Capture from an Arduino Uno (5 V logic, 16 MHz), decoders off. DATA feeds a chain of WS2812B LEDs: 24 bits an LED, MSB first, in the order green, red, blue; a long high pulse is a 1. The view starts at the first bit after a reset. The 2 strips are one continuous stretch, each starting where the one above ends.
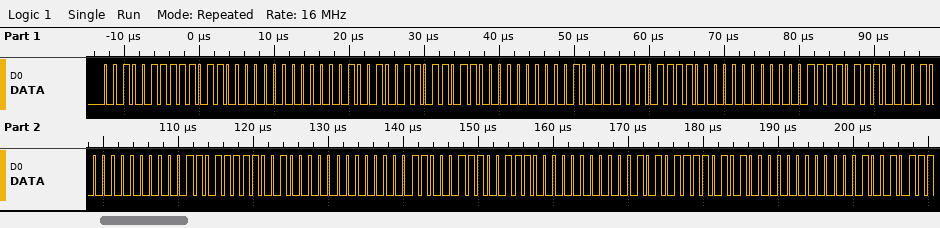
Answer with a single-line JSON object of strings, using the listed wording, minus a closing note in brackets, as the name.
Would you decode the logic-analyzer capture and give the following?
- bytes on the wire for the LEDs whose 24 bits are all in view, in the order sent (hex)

{"bytes on the wire for the LEDs whose 24 bits are all in view, in the order sent": "27 D8 00 24 DB 00 21 DE 00 1E E1 00 1B E4 00 18 E7 00 15 EA 00"}
